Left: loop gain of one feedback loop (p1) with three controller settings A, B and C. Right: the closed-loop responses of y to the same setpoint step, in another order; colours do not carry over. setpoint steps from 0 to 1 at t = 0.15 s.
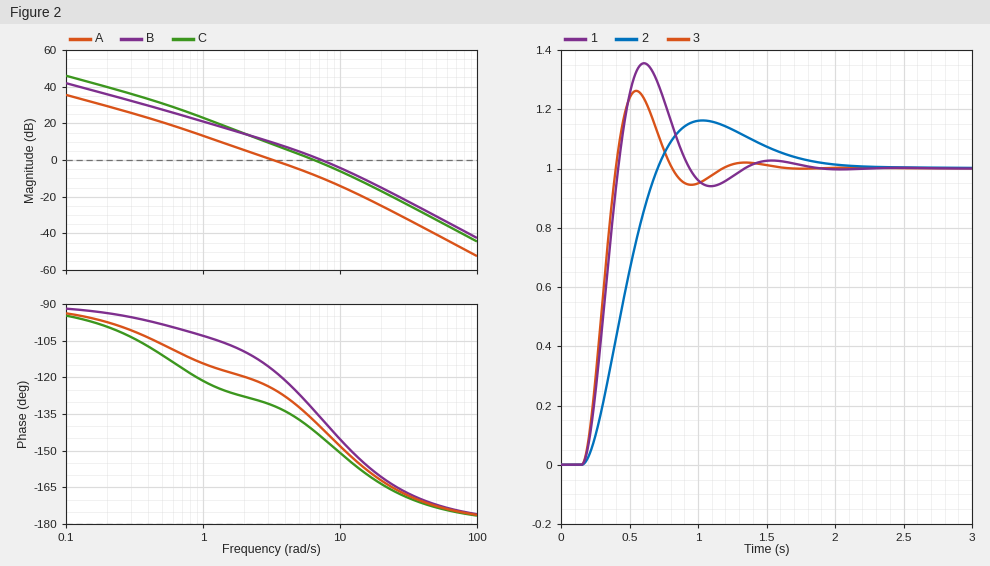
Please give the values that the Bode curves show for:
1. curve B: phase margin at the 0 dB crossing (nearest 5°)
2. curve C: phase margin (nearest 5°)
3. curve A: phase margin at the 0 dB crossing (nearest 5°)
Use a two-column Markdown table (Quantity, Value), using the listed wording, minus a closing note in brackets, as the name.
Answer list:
| Quantity | Value |
|---|---|
| curve B: phase margin at the 0 dB crossing | 45° |
| curve C: phase margin | 40° |
| curve A: phase margin at the 0 dB crossing | 55° |
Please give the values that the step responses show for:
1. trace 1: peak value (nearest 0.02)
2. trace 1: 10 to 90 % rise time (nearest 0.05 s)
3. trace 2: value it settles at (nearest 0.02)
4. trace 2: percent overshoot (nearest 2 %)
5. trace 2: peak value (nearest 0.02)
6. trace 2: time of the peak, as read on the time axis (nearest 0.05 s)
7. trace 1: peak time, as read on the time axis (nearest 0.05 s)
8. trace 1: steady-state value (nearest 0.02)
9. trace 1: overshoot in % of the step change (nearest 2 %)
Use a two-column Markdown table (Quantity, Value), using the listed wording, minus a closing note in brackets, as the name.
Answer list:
| Quantity | Value |
|---|---|
| trace 1: peak value | 1.36 |
| trace 1: 10 to 90 % rise time | 0.20 s |
| trace 2: value it settles at | 1.00 |
| trace 2: percent overshoot | 16 % |
| trace 2: peak value | 1.16 |
| trace 2: time of the peak, as read on the time axis | 1.05 s |
| trace 1: peak time, as read on the time axis | 0.60 s |
| trace 1: steady-state value | 1.00 |
| trace 1: overshoot in % of the step change | 36 % |
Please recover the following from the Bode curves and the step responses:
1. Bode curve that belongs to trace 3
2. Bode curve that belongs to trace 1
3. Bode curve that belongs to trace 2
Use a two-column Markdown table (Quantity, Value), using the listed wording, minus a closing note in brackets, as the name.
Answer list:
| Quantity | Value |
|---|---|
| Bode curve that belongs to trace 3 | B |
| Bode curve that belongs to trace 1 | C |
| Bode curve that belongs to trace 2 | A |
